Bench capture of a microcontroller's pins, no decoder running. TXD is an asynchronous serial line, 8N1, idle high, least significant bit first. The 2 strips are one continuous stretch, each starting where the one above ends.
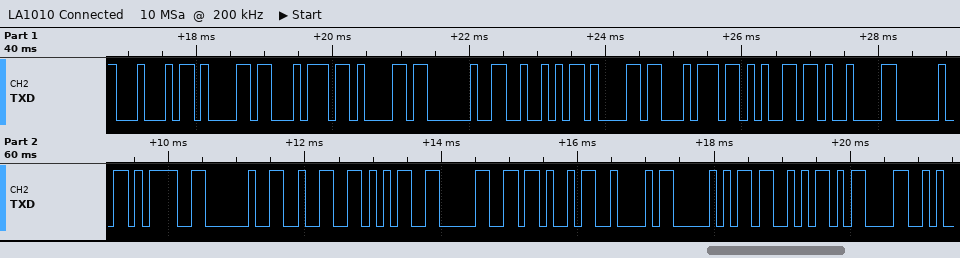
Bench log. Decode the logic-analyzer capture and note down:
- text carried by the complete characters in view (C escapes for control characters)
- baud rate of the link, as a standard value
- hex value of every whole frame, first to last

"Data Rate\t = 250KBPS\r"
9600 baud
44 61 74 61 20 52 61 74 65 09 20 3D 20 32 35 30 4B 42 50 53 0D
